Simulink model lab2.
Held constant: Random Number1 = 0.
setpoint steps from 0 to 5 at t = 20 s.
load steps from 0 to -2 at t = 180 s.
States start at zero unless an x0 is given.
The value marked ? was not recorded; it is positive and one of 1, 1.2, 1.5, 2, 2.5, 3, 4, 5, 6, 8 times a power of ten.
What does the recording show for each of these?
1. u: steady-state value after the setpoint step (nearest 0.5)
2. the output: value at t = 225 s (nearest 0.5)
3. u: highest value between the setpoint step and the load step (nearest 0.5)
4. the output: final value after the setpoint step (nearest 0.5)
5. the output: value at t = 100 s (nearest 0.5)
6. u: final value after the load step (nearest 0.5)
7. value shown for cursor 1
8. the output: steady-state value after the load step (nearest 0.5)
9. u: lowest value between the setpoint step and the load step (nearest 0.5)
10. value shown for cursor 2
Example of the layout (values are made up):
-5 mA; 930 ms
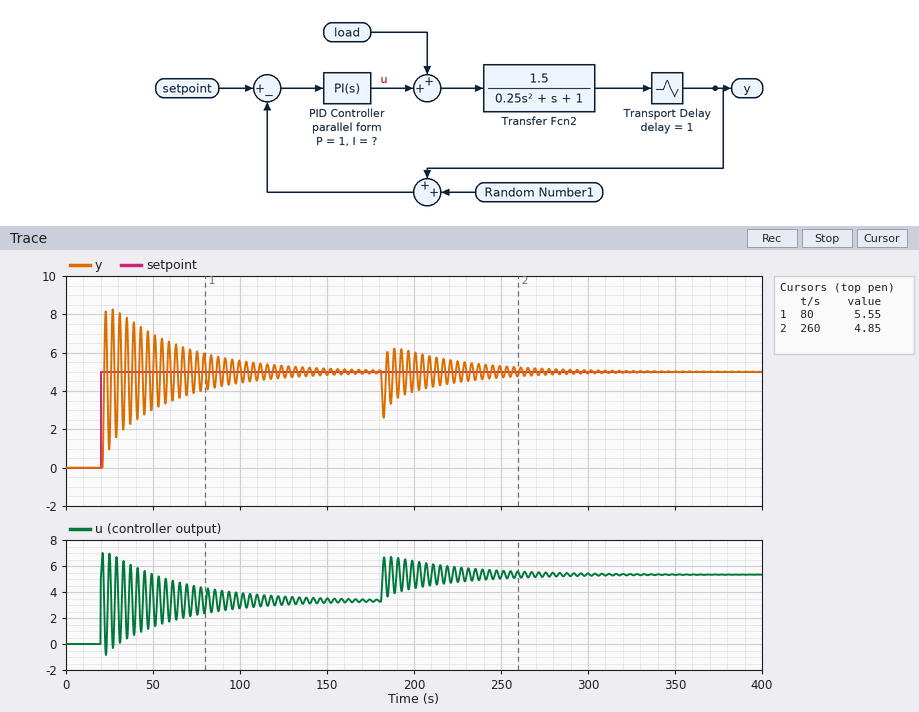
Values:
3.5; 5.5; 7.0; 5.0; 5.5; 5.5; 5.55; 5.0; -1.0; 4.85
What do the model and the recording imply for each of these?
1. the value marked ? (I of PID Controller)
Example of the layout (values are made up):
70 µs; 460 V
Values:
0.4
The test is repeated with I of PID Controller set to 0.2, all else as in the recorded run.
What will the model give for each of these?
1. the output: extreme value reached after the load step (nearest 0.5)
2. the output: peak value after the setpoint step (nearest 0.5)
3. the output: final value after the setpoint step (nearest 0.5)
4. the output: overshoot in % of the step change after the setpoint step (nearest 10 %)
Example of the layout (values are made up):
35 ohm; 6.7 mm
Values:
2.5; 7.0; 5.0; 40 %
